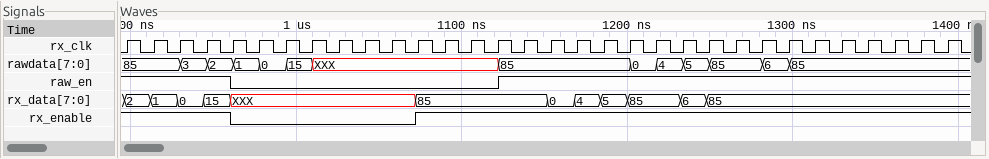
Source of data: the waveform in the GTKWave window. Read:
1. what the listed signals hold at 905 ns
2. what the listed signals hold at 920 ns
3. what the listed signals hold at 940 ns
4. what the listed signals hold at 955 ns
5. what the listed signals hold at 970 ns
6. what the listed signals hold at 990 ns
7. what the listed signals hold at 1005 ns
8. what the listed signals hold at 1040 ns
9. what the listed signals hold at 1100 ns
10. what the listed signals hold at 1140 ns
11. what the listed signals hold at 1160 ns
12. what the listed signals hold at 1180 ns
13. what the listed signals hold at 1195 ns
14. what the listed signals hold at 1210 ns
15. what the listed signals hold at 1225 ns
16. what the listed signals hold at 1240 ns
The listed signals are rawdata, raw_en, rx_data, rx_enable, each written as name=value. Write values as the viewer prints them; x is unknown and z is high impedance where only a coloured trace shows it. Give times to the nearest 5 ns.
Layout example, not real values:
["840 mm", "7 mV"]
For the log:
["rawdata=85, raw_en=1, rx_data=2, rx_enable=1", "rawdata=85, raw_en=1, rx_data=1, rx_enable=1", "rawdata=3, raw_en=1, rx_data=0, rx_enable=1", "rawdata=2, raw_en=1, rx_data=15, rx_enable=1", "rawdata=1, raw_en=0, rx_data=XXX, rx_enable=0", "rawdata=0, raw_en=0, rx_data=XXX, rx_enable=0", "rawdata=15, raw_en=0, rx_data=XXX, rx_enable=0", "rawdata=XXX, raw_en=0, rx_data=XXX, rx_enable=0", "rawdata=XXX, raw_en=0, rx_data=85, rx_enable=1", "rawdata=85, raw_en=1, rx_data=85, rx_enable=1", "rawdata=85, raw_en=1, rx_data=0, rx_enable=1", "rawdata=85, raw_en=1, rx_data=4, rx_enable=1", "rawdata=85, raw_en=1, rx_data=5, rx_enable=1", "rawdata=0, raw_en=1, rx_data=85, rx_enable=1", "rawdata=4, raw_en=1, rx_data=85, rx_enable=1", "rawdata=5, raw_en=1, rx_data=6, rx_enable=1"]
